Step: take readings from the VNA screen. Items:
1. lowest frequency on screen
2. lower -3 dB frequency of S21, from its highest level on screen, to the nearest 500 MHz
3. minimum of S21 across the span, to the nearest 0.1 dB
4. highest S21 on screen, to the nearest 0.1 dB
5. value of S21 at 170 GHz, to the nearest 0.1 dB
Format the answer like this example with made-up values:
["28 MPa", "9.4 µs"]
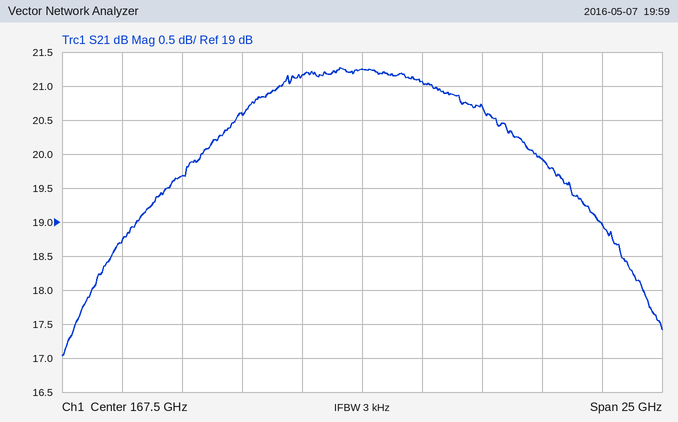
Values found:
["155 GHz", "156.5 GHz", "17.0 dB", "21.3 dB", "21.1 dB"]
